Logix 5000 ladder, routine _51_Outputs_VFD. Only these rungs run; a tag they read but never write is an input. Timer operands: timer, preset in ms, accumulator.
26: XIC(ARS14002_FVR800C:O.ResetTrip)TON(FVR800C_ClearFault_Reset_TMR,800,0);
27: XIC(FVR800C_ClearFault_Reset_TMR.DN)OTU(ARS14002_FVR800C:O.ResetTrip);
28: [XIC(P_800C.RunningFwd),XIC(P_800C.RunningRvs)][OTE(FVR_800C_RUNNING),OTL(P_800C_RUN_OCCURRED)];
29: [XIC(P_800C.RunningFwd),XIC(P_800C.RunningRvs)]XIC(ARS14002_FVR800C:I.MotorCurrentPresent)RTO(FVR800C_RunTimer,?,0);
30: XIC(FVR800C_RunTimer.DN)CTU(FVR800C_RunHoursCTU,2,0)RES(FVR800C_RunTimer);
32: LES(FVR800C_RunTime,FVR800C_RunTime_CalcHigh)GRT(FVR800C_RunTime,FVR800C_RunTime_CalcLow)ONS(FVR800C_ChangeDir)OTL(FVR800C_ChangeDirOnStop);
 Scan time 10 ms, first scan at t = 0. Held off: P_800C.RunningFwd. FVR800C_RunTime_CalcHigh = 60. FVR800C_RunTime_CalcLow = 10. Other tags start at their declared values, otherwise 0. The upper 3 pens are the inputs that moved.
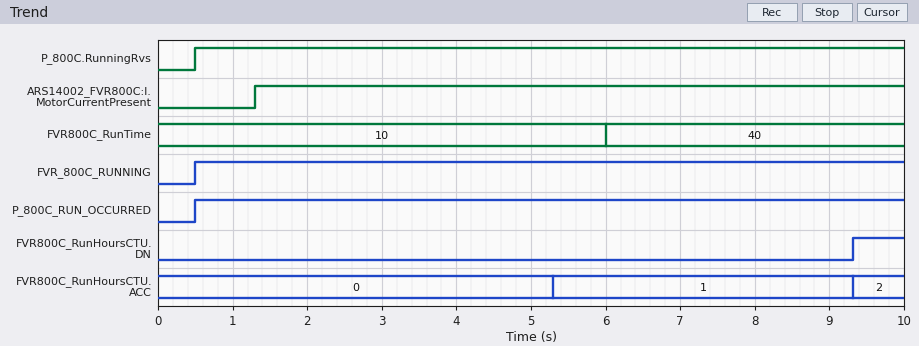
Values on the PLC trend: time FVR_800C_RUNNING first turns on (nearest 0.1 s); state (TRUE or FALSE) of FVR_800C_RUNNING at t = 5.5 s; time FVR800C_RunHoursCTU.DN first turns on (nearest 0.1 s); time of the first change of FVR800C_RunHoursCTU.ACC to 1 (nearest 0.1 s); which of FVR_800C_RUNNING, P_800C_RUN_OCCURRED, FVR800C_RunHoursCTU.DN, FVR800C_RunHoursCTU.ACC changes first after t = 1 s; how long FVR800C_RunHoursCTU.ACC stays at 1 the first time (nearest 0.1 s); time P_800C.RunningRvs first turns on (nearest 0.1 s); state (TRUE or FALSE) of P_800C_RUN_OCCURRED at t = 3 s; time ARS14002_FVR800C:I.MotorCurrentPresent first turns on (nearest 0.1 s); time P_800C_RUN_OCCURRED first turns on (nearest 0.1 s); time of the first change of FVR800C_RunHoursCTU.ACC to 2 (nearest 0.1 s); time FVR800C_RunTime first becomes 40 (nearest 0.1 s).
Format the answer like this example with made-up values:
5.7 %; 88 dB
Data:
0.5 s; TRUE; 9.3 s; 5.3 s; FVR800C_RunHoursCTU.ACC; 4.0 s; 0.5 s; TRUE; 1.3 s; 0.5 s; 9.3 s; 6.0 s
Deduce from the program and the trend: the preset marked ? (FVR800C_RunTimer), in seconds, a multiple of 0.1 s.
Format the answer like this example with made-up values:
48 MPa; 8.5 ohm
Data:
4.0 s
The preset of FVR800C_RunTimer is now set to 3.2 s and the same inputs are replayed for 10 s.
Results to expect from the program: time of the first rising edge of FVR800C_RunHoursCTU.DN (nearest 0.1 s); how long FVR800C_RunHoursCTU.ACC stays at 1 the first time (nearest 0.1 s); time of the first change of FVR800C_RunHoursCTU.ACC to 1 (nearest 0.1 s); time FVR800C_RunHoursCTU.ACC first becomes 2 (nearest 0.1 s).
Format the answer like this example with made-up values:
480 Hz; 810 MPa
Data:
7.7 s; 3.2 s; 4.5 s; 7.7 s
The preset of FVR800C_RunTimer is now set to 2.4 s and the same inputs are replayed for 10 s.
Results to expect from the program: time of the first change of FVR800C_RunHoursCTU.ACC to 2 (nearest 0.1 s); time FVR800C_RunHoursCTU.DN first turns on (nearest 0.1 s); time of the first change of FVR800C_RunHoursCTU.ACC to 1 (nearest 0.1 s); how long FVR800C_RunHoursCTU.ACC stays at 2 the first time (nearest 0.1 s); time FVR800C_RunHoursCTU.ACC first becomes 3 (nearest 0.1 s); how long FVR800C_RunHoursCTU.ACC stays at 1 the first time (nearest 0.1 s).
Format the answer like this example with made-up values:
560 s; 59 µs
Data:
6.1 s; 6.1 s; 3.7 s; 2.4 s; 8.5 s; 2.4 s
